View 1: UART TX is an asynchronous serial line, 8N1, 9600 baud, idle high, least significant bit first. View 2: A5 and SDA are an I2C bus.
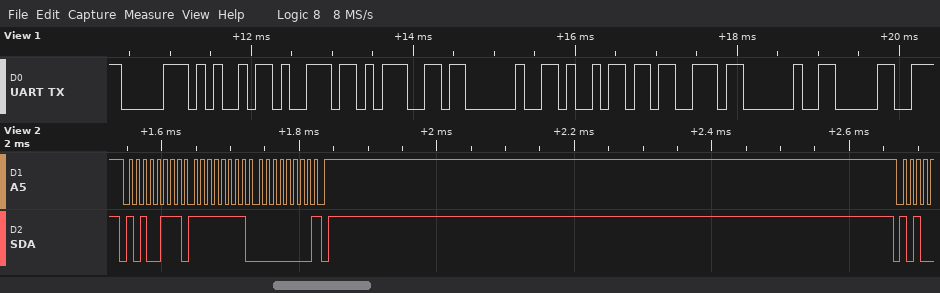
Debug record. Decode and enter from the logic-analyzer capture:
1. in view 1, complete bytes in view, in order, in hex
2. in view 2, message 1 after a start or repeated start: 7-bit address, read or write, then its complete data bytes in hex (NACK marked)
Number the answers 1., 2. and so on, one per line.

1. 70 69 6E 67 20 69 73 20 30
2. 0x53 read: FF 00 NACK
